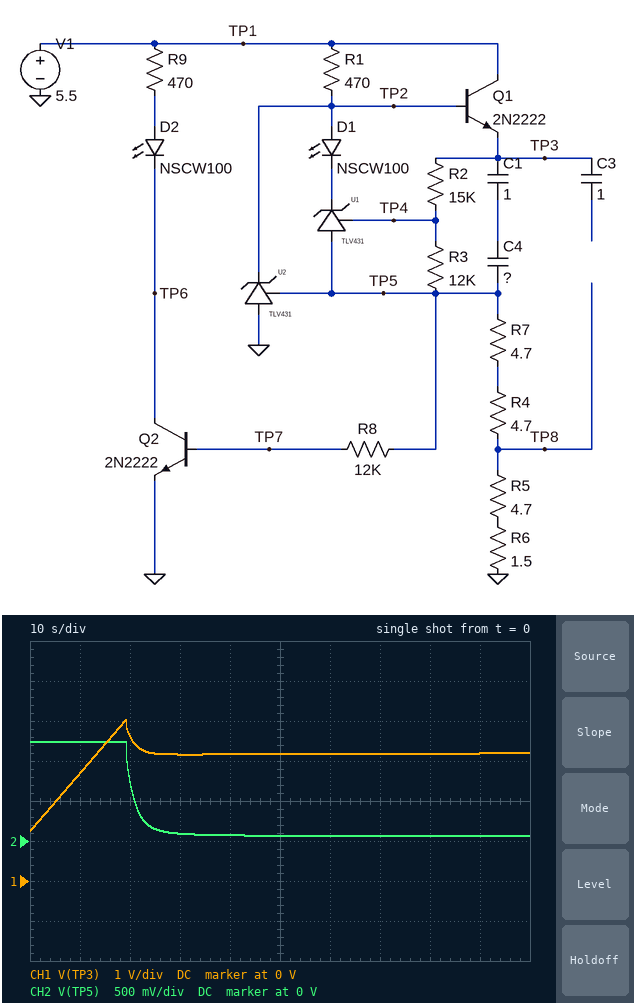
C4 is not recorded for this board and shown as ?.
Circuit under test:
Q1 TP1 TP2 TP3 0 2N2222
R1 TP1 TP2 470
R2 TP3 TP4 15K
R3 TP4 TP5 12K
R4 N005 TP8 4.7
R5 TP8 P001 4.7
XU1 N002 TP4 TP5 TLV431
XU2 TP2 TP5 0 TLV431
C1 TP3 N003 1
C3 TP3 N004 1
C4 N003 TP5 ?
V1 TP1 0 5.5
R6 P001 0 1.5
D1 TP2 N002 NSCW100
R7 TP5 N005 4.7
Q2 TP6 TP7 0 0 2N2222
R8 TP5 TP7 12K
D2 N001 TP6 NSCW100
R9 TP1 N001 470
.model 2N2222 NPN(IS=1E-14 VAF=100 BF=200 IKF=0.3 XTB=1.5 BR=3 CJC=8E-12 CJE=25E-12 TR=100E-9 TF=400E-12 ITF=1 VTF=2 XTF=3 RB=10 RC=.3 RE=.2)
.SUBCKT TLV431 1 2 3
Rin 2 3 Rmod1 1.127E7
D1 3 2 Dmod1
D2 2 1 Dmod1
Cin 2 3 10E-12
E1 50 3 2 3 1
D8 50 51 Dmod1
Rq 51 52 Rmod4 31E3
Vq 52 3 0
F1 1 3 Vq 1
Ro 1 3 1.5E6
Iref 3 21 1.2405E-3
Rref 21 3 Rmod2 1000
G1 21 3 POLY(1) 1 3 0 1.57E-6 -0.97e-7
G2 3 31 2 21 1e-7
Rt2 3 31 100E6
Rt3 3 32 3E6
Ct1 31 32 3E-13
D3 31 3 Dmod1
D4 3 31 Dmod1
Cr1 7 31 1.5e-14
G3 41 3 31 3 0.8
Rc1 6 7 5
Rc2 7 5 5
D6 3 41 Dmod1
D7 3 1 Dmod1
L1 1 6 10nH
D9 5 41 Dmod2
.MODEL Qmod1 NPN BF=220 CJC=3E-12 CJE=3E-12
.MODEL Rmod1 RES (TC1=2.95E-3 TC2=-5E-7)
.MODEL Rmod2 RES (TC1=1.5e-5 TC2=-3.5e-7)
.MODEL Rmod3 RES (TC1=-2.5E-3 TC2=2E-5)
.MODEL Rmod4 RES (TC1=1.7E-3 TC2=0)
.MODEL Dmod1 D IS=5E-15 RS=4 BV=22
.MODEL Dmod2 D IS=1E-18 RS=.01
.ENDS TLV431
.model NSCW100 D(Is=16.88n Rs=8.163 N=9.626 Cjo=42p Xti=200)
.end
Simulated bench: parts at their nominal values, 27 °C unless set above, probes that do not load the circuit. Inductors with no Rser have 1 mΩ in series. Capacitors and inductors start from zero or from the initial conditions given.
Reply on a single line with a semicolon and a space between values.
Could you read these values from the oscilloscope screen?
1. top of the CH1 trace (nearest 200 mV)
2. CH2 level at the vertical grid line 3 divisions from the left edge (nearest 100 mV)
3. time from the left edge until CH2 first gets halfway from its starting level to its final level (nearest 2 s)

4.0 V; 100 mV; 20 s
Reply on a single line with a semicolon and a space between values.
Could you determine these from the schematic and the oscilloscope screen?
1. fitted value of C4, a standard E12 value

1.2 F
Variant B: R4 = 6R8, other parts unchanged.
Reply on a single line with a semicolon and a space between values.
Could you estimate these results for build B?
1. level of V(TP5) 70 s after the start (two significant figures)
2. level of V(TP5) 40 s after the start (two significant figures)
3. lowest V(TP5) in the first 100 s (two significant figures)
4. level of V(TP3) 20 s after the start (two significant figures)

70 mV; 84 mV; 68 mV; 3.8 V
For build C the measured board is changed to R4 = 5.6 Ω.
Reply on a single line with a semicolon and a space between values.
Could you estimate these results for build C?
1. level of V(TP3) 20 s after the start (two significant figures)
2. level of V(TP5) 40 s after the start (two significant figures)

4.0 V; 76 mV
